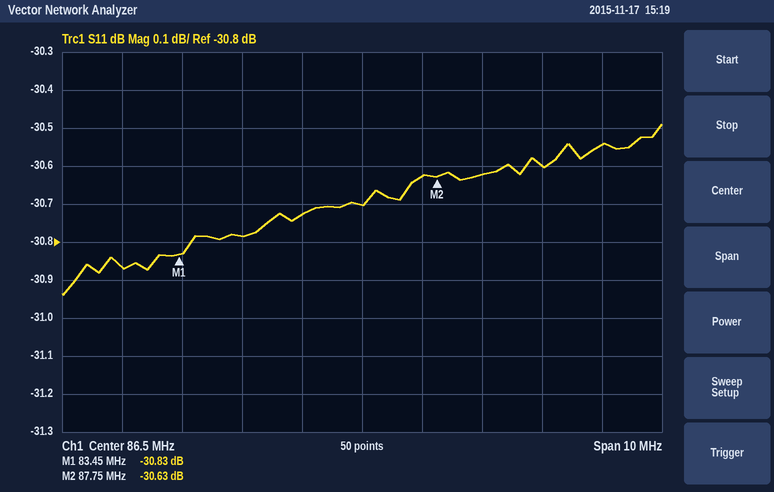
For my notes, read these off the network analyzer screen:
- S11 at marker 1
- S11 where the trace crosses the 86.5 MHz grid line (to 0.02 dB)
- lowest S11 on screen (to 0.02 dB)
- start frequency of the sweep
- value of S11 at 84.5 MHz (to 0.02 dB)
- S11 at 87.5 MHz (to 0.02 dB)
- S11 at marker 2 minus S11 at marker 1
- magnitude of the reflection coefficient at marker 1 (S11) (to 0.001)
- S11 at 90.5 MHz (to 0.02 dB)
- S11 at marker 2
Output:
-30.83 dB
-30.70 dB
-30.94 dB
81.5 MHz
-30.78 dB
-30.62 dB
0.20 dB
0.029
-30.54 dB
-30.63 dB
